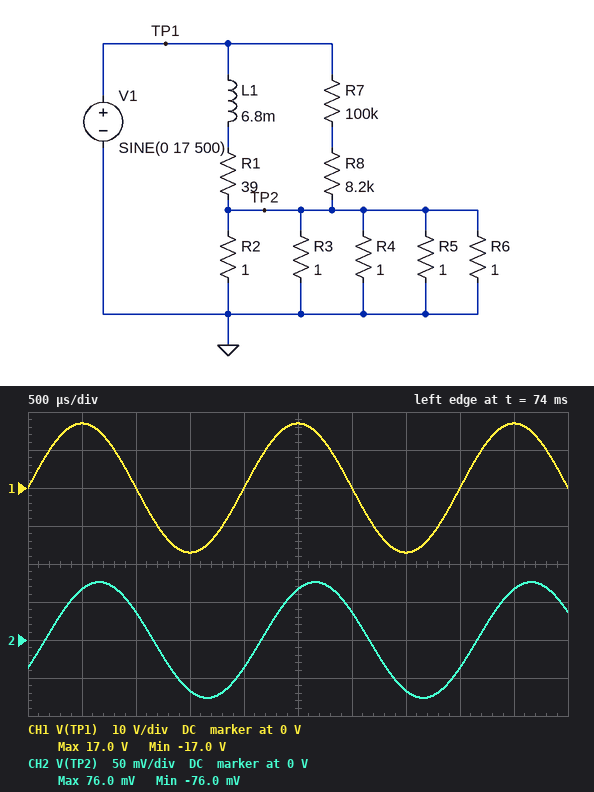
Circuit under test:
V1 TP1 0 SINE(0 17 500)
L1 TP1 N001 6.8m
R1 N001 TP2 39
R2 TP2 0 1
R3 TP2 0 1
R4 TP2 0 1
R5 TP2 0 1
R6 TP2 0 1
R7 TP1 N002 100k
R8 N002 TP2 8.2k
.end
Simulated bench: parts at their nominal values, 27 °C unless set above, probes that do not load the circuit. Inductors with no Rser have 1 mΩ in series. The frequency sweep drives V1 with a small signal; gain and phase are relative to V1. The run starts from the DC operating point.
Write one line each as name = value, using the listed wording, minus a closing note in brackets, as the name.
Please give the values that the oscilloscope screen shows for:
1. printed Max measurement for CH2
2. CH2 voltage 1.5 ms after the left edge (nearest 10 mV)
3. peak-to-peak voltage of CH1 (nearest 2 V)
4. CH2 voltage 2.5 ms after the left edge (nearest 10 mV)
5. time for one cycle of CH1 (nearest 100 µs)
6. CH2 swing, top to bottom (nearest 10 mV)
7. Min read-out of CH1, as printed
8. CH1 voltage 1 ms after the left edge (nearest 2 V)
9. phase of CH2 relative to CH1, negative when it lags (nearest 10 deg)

printed Max measurement for CH2 = 76.0 mV
CH2 voltage 1.5 ms after the left edge = -70 mV
peak-to-peak voltage of CH1 = 34 V
CH2 voltage 2.5 ms after the left edge = 70 mV
time for one cycle of CH1 = 2.0 ms
CH2 swing, top to bottom = 150 mV
Min read-out of CH1, as printed = -17.0 V
CH1 voltage 1 ms after the left edge = 0 V
phase of CH2 relative to CH1, negative when it lags = -30 deg
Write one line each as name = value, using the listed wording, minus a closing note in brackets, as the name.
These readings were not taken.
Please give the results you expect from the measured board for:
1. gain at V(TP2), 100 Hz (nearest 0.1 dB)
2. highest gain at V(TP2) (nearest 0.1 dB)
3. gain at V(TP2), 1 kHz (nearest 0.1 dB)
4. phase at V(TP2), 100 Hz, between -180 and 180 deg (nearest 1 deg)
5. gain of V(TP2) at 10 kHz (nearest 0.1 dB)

gain at V(TP2), 100 Hz = -45.9 dB
highest gain at V(TP2) = -45.8 dB
gain at V(TP2), 1 kHz = -49.2 dB
phase at V(TP2), 100 Hz, between -180 and 180 deg = -6 deg
gain of V(TP2) at 10 kHz = -66.6 dB
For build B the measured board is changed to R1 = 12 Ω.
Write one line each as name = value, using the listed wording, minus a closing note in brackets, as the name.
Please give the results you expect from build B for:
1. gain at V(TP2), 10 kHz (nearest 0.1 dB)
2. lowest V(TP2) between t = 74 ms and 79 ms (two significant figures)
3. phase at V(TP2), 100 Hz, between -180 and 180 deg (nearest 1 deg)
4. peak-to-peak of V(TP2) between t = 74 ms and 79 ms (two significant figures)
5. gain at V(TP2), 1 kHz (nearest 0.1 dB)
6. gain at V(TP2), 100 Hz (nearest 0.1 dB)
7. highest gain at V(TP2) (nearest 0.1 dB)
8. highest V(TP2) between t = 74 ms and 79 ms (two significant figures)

gain at V(TP2), 10 kHz = -66.6 dB
lowest V(TP2) between t = 74 ms and 79 ms = -140 mV
phase at V(TP2), 100 Hz, between -180 and 180 deg = -19 deg
peak-to-peak of V(TP2) between t = 74 ms and 79 ms = 280 mV
gain at V(TP2), 1 kHz = -46.9 dB
gain at V(TP2), 100 Hz = -36.2 dB
highest gain at V(TP2) = -35.7 dB
highest V(TP2) between t = 74 ms and 79 ms = 140 mV
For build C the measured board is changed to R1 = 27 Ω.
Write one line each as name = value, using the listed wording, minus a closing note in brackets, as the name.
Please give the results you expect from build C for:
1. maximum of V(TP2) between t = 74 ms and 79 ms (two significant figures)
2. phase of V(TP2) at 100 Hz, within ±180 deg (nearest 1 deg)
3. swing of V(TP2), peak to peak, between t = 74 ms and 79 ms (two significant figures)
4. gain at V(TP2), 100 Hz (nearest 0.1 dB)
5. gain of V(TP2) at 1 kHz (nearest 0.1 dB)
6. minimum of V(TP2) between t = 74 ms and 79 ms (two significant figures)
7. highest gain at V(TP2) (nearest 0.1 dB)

maximum of V(TP2) between t = 74 ms and 79 ms = 98 mV
phase of V(TP2) at 100 Hz, within ±180 deg = -9 deg
swing of V(TP2), peak to peak, between t = 74 ms and 79 ms = 200 mV
gain at V(TP2), 100 Hz = -42.8 dB
gain of V(TP2) at 1 kHz = -48.1 dB
minimum of V(TP2) between t = 74 ms and 79 ms = -98 mV
highest gain at V(TP2) = -42.7 dB
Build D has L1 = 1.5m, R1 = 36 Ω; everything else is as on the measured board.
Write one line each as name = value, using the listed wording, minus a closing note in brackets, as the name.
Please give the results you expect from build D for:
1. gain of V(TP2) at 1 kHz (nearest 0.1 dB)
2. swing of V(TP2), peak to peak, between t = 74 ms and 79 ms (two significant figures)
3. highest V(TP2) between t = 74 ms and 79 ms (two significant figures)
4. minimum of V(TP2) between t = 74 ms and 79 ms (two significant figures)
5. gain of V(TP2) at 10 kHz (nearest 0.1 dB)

gain of V(TP2) at 1 kHz = -45.4 dB
swing of V(TP2), peak to peak, between t = 74 ms and 79 ms = 190 mV
highest V(TP2) between t = 74 ms and 79 ms = 93 mV
minimum of V(TP2) between t = 74 ms and 79 ms = -93 mV
gain of V(TP2) at 10 kHz = -54.1 dB
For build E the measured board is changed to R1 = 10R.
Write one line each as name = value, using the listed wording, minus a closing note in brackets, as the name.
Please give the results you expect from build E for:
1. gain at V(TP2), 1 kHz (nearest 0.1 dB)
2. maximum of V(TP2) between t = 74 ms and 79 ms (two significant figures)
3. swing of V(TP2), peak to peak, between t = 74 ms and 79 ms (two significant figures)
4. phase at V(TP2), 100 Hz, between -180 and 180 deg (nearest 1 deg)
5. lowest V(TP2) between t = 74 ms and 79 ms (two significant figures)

gain at V(TP2), 1 kHz = -46.8 dB
maximum of V(TP2) between t = 74 ms and 79 ms = 140 mV
swing of V(TP2), peak to peak, between t = 74 ms and 79 ms = 290 mV
phase at V(TP2), 100 Hz, between -180 and 180 deg = -23 deg
lowest V(TP2) between t = 74 ms and 79 ms = -140 mV
